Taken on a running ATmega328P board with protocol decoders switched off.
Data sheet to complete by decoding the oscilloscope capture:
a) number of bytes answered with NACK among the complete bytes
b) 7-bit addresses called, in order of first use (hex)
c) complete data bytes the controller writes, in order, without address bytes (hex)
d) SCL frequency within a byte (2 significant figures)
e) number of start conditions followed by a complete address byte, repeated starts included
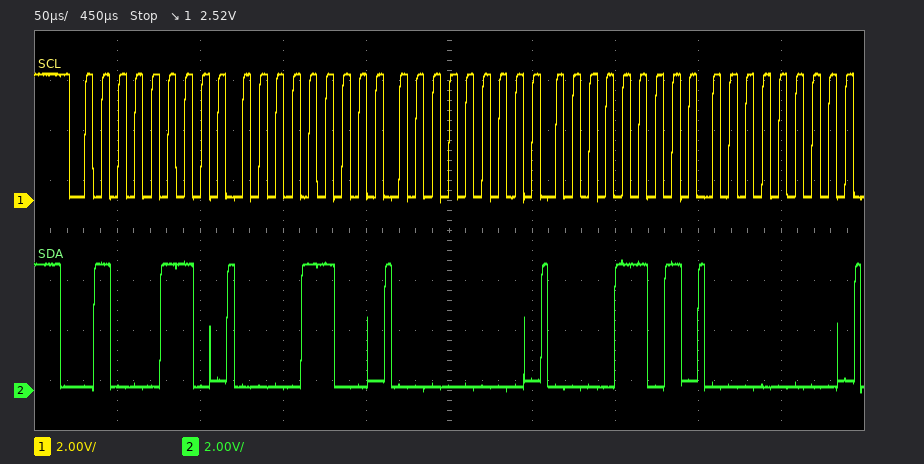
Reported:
0
0x23
0C 00 0D 00
100 kHz
1
